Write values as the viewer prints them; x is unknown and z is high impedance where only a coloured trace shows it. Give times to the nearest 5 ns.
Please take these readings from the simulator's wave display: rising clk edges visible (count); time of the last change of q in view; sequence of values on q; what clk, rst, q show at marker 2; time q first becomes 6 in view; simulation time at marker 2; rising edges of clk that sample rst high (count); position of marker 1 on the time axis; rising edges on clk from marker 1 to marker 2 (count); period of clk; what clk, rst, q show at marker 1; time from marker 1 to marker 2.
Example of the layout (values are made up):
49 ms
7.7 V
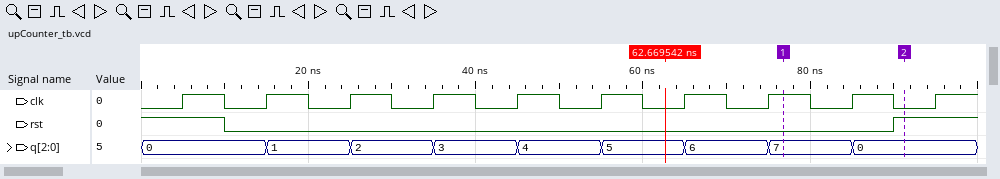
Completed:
10
85 ns
0, 1, 2, 3, 4, 5, 6, 7, 0
clk=0, rst=1, q=0
65 ns
90 ns
2
75 ns
1
10 ns
clk=1, rst=0, q=7
15 ns
